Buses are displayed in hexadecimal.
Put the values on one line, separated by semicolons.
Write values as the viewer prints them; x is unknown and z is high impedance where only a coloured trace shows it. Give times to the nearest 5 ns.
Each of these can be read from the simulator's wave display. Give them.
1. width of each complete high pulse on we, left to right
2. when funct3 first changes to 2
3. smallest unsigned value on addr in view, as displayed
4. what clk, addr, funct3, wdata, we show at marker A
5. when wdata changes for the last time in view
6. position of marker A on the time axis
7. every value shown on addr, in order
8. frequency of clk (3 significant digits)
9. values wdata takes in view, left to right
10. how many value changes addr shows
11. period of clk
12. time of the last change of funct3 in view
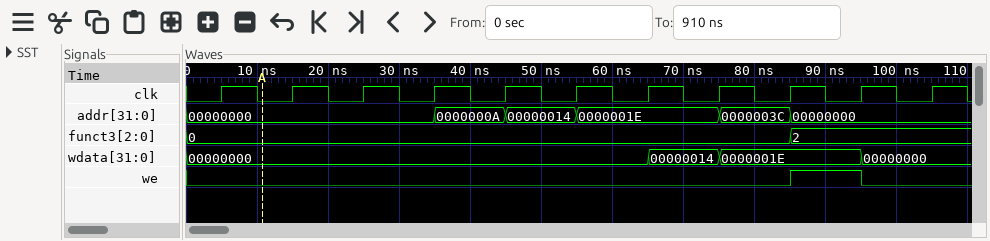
10 ns; 85 ns; 00000000; clk=0, addr=00000000, funct3=0, wdata=00000000, we=0; 95 ns; 10 ns; 00000000, 0000000A, 00000014, 0000001E, 0000003C, 00000000; 100 MHz; 00000000, 00000014, 0000001E, 00000000; 5; 10 ns; 85 ns
